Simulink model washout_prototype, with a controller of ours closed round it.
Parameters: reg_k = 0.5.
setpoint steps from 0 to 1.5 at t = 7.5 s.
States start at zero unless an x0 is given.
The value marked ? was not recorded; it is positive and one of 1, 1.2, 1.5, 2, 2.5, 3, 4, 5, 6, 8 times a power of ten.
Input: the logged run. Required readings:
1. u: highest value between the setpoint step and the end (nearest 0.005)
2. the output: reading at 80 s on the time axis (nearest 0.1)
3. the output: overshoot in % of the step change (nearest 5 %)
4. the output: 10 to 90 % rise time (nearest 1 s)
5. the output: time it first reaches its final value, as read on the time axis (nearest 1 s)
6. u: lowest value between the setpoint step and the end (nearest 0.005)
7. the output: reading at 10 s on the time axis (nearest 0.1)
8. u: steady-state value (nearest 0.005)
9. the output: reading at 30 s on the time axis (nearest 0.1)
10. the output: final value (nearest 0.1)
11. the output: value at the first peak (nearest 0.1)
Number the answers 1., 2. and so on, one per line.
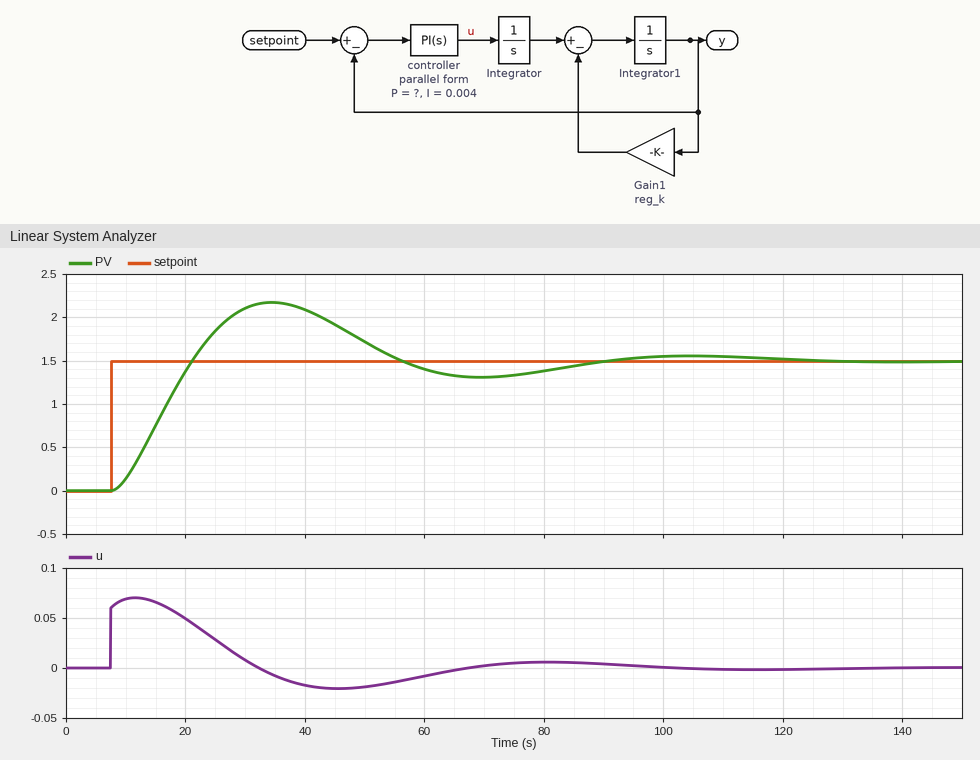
1. 0.070
2. 1.4
3. 45 %
4. 10 s
5. 21 s
6. -0.020
7. 0.1
8. 0.000
9. 2.1
10. 1.5
11. 2.2
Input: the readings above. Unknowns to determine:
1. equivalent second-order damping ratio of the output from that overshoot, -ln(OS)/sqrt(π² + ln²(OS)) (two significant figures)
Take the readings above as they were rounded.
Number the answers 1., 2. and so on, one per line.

1. 0.25
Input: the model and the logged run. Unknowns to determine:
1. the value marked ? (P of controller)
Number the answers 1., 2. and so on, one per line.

1. 0.04
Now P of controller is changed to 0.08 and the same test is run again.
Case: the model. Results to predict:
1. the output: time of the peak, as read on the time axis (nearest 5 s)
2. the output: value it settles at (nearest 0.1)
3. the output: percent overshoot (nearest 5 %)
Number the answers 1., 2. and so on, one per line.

1. 25 s
2. 1.5
3. 25 %
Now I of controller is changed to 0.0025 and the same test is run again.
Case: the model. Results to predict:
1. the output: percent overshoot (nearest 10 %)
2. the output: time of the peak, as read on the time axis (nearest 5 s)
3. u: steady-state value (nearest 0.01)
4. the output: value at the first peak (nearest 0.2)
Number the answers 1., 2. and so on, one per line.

1. 30 %
2. 40 s
3. 0.00
4. 2.0
